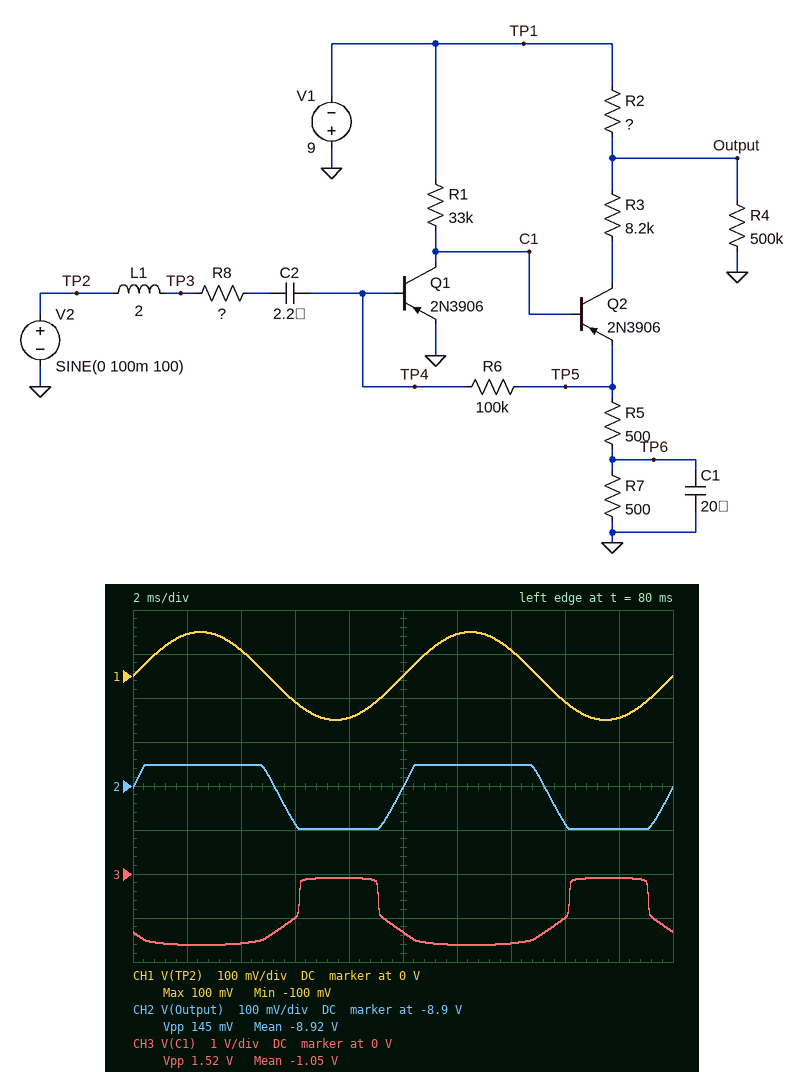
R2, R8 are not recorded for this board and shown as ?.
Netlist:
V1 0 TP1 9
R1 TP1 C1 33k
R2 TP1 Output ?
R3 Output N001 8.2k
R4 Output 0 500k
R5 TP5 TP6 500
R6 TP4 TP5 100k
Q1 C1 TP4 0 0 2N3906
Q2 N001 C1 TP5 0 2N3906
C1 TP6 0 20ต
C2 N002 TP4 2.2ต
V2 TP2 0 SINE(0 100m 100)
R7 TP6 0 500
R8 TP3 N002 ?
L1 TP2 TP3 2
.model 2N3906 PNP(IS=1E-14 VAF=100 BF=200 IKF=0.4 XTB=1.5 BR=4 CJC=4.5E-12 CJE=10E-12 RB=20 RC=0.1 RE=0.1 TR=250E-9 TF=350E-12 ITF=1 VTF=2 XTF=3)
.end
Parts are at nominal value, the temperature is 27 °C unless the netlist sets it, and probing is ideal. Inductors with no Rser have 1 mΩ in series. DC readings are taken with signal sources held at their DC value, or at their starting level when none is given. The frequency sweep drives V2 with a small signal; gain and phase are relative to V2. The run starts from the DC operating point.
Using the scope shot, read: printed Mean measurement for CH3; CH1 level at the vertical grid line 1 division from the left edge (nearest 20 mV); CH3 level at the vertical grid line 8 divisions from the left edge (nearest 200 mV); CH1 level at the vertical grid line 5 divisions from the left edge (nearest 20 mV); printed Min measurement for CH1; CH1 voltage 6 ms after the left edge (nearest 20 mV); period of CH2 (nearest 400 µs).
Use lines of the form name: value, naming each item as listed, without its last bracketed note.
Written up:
printed Mean measurement for CH3: -1.05 V
CH1 level at the vertical grid line 1 division from the left edge: 100 mV
CH3 level at the vertical grid line 8 divisions from the left edge: -1.0 V
CH1 level at the vertical grid line 5 divisions from the left edge: 0 V
printed Min measurement for CH1: -100 mV
CH1 voltage 6 ms after the left edge: -60 mV
period of CH2: 10.0 ms
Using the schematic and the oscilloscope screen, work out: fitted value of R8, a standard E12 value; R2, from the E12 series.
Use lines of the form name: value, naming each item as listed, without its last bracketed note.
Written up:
fitted value of R8, a standard E12 value: 15 kΩ
R2, from the E12 series: 150 Ω
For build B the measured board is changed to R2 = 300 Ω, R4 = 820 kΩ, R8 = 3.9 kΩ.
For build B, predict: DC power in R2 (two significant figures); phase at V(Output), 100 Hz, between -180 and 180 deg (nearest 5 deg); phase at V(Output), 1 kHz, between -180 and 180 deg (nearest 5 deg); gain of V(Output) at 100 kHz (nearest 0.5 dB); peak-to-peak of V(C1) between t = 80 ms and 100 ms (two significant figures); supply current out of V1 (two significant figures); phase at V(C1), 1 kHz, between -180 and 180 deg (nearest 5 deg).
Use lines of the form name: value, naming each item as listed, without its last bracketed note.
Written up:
DC power in R2: 160 µW
phase at V(Output), 100 Hz, between -180 and 180 deg: -15 deg
phase at V(Output), 1 kHz, between -180 and 180 deg: -70 deg
gain of V(Output) at 100 kHz: -27.0 dB
peak-to-peak of V(C1) between t = 80 ms and 100 ms: 1.6 V
supply current out of V1: 970 µA
phase at V(C1), 1 kHz, between -180 and 180 deg: 110 deg
